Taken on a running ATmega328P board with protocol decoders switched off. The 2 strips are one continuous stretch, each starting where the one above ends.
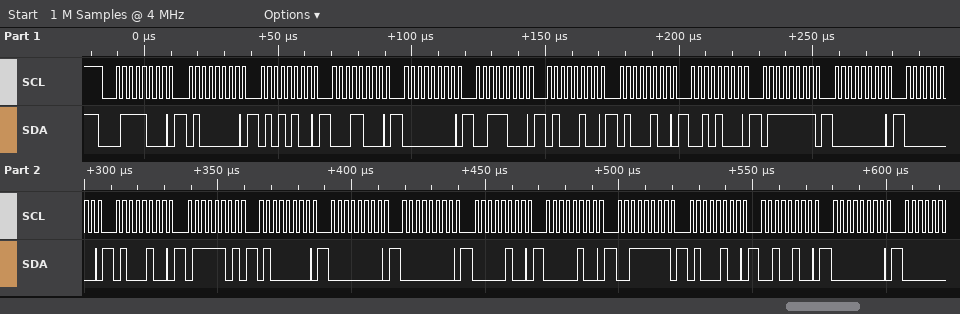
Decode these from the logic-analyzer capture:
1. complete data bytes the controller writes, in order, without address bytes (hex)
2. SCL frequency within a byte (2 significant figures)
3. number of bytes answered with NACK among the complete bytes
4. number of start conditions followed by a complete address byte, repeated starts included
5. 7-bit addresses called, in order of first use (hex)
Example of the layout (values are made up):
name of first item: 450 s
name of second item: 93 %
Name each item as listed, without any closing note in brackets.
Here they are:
complete data bytes the controller writes, in order, without address bytes: 40 54 18 00 38 44 44 28 7F 00 00 44 7D 40 00 00 04 04 3F 44 24 00
SCL frequency within a byte: 400 kHz
number of bytes answered with NACK among the complete bytes: 0
number of start conditions followed by a complete address byte, repeated starts included: 1
7-bit addresses called, in order of first use: 0x3C
